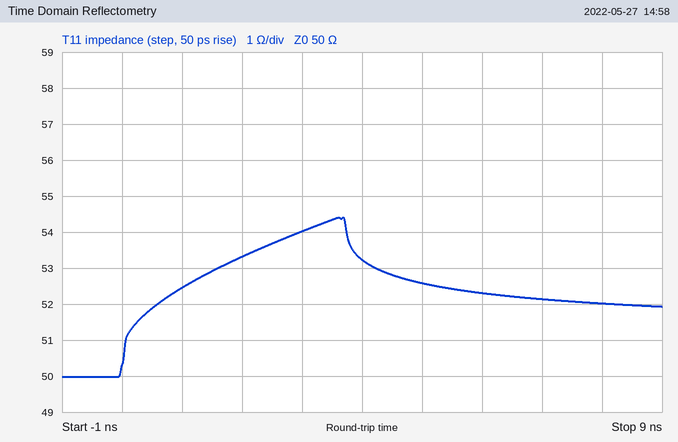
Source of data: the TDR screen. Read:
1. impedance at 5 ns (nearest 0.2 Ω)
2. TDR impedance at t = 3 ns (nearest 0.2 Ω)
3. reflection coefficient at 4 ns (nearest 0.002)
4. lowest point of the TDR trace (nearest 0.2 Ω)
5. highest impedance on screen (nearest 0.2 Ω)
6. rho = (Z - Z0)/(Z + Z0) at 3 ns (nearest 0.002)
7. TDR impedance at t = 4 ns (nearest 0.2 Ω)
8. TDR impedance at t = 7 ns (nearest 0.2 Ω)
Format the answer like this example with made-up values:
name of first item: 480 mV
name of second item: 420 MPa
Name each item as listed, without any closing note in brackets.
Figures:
impedance at 5 ns: 52.6 Ω
TDR impedance at t = 3 ns: 54.0 Ω
reflection coefficient at 4 ns: +0.032
lowest point of the TDR trace: 50.0 Ω
highest impedance on screen: 54.4 Ω
rho = (Z - Z0)/(Z + Z0) at 3 ns: +0.038
TDR impedance at t = 4 ns: 53.2 Ω
TDR impedance at t = 7 ns: 52.2 Ω
